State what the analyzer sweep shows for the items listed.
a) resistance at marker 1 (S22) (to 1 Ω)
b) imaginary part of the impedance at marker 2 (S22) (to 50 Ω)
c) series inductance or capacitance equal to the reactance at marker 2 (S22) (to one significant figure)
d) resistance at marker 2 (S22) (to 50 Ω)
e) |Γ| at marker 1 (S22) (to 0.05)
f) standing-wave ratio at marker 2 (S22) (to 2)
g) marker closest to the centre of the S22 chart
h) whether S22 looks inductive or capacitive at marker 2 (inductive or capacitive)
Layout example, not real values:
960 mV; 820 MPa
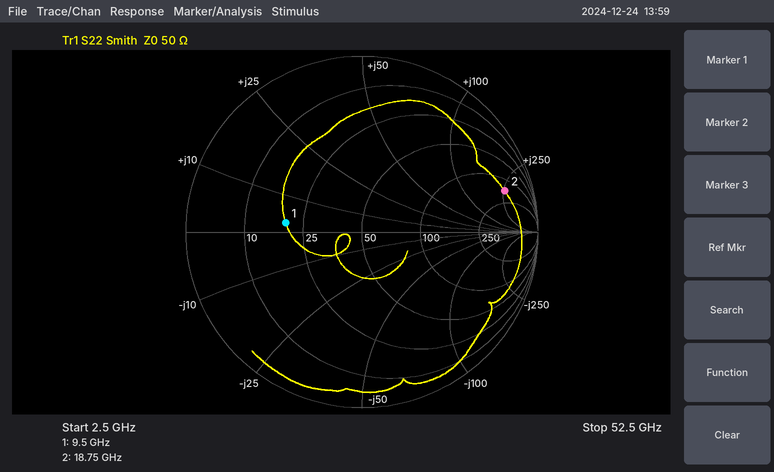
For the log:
20 Ω; +250 Ω; 2 nH; 150 Ω; 0.45; 12; marker 1; inductive
